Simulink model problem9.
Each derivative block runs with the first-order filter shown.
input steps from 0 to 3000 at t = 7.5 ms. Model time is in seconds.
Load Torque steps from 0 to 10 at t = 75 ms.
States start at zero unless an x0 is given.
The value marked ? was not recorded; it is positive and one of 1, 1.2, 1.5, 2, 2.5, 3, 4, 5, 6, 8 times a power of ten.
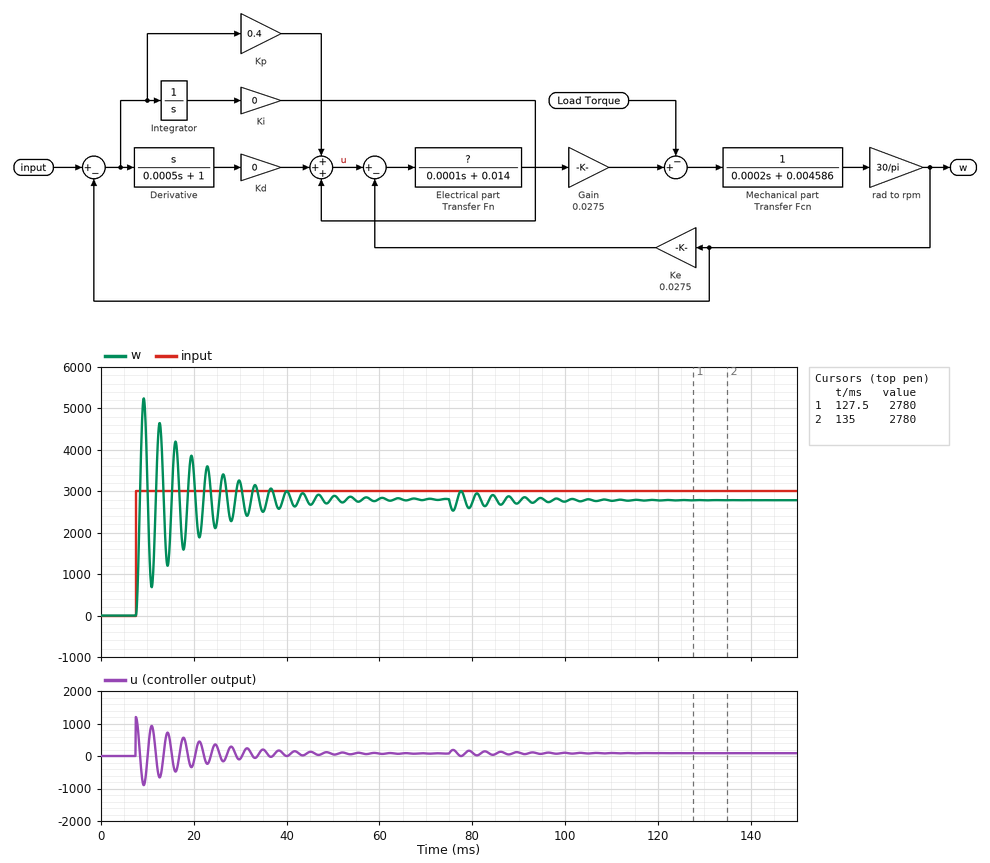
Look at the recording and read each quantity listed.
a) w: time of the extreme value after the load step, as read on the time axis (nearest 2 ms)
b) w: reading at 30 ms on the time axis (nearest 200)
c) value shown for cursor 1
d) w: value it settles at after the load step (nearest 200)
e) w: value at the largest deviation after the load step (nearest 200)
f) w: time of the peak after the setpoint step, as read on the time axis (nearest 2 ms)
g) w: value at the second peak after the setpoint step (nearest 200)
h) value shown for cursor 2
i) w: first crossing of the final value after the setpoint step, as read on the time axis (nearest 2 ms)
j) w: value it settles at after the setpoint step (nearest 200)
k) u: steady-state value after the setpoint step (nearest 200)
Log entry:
76 ms
3200
2780
2800
2600
10 ms
4600
2780
8 ms
2800
0
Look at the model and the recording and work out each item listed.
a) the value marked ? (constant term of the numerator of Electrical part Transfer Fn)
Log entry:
0.6
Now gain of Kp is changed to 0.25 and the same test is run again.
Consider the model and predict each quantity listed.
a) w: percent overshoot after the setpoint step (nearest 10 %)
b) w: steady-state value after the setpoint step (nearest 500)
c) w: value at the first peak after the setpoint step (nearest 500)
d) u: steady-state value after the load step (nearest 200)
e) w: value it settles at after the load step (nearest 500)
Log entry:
80 %
2500
5000
0
2500
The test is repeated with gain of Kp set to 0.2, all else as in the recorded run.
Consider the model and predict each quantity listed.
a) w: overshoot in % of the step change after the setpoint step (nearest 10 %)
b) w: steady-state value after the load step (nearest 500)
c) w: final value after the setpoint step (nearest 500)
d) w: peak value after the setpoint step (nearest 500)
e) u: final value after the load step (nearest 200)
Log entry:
80 %
2500
2500
5000
0
